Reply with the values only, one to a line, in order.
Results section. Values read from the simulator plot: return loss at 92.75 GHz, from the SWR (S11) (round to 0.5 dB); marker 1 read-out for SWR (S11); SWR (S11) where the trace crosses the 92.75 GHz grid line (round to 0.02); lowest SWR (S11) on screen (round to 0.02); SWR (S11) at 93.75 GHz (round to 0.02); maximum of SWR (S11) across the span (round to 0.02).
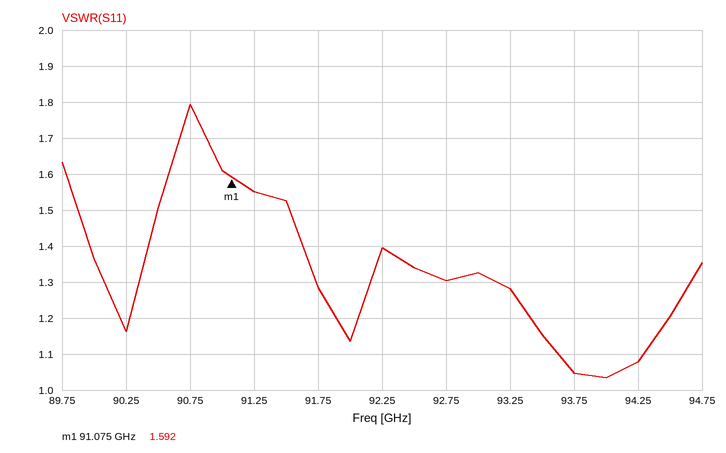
17.5 dB
1.592
1.30
1.04
1.04
1.80
